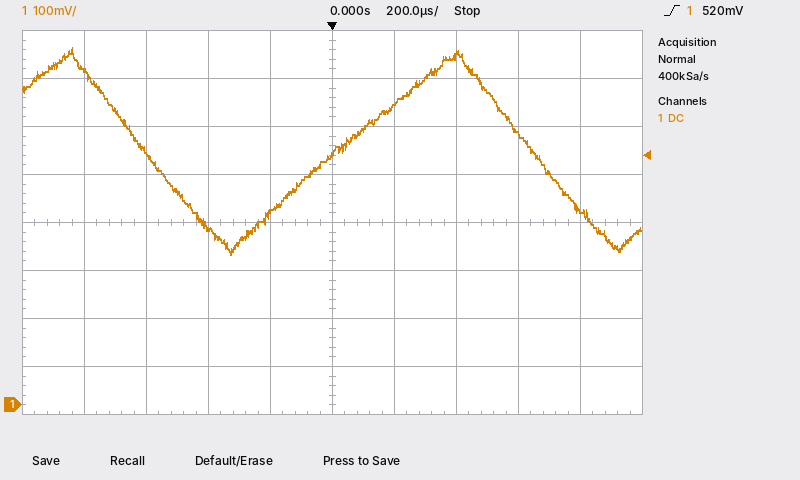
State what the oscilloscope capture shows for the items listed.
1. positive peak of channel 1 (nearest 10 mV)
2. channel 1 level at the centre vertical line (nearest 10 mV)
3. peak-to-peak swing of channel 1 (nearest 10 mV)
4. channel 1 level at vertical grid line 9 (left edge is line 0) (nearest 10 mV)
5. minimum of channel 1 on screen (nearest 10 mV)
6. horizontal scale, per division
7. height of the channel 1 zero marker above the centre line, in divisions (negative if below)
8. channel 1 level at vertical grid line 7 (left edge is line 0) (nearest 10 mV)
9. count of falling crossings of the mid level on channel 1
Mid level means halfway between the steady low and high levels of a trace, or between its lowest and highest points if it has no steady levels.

740 mV
520 mV
430 mV
410 mV
310 mV
200 µs
-3.8 div
730 mV
2
